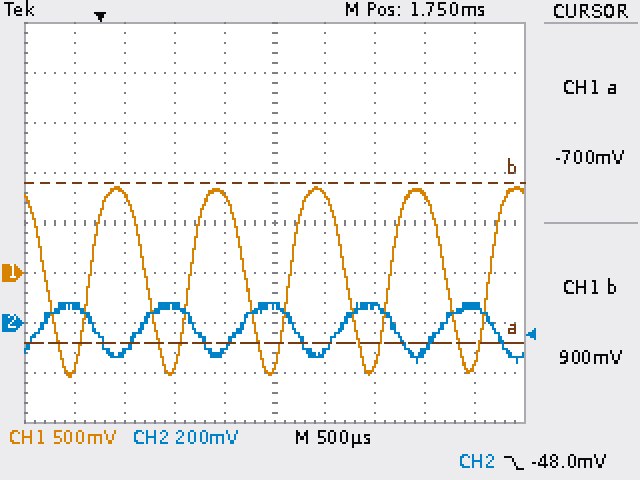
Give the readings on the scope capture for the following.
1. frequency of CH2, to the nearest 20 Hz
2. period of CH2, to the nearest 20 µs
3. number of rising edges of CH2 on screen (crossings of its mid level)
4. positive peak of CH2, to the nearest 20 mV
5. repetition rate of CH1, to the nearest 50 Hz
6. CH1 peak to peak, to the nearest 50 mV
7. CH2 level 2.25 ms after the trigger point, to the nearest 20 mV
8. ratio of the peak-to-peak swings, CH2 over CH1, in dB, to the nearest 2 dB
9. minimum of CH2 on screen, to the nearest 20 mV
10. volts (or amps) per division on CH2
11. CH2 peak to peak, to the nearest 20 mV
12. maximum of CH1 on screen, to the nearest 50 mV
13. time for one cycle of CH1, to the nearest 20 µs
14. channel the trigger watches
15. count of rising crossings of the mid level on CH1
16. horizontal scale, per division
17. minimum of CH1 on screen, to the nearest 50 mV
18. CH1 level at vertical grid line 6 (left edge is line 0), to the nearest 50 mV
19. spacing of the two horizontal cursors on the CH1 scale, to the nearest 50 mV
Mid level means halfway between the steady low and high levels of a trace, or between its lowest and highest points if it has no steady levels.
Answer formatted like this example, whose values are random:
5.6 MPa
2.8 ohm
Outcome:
1.00 kHz
1.00 ms
5
80 mV
1.00 kHz
1.90 V
-120 mV
-18 dB
-160 mV
200 mV
240 mV
850 mV
1.00 ms
CH2
5
500 µs
-1.05 V
800 mV
1.60 V
